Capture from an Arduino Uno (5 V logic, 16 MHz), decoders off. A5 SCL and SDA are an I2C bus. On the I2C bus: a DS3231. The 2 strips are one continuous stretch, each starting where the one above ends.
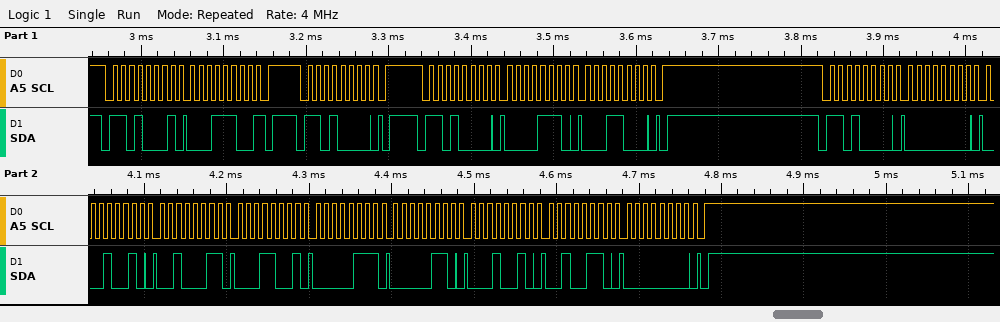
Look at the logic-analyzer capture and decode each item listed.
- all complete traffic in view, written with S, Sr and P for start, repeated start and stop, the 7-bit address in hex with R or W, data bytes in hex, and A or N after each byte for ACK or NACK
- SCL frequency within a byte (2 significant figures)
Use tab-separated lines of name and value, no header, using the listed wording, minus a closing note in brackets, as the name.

all complete traffic in view, written with S, Sr and P for start, repeated start and stop, the 7-bit address in hex with R or W, data bytes in hex, and A or N after each byte for ACK or NACK	S 68R A 1C N P S 68W A P S 68W A 0E A 18 A P S 68W A 00 A 12 A 23 A 19 A 07 A 06 A 12 A 26 A 00 A P
SCL frequency within a byte	100 kHz
